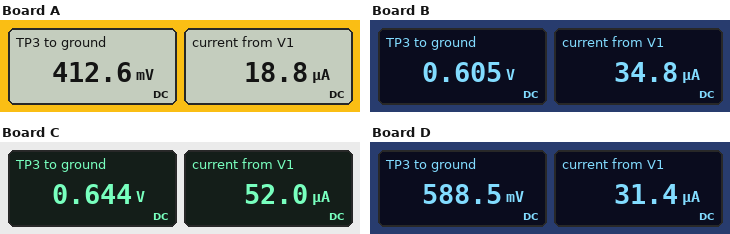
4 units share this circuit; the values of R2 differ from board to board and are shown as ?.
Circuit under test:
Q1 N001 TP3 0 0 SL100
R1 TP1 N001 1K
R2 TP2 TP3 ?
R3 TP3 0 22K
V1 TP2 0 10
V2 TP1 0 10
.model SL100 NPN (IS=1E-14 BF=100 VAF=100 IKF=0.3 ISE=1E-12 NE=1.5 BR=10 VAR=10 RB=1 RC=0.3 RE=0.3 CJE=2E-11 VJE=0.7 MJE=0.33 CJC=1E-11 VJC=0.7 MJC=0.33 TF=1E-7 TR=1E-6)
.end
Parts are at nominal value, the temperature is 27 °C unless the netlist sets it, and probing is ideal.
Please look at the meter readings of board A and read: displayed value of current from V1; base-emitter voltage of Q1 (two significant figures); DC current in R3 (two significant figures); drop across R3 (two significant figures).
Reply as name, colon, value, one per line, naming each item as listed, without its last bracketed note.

displayed value of current from V1: 18.8 µA
base-emitter voltage of Q1: 410 mV
DC current in R3: 19 µA
drop across R3: 410 mV
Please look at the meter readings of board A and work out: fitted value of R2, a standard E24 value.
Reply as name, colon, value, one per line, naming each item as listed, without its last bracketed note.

fitted value of R2, a standard E24 value: 510 kΩ
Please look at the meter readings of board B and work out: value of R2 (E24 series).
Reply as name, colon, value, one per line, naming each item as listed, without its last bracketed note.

value of R2: 270 kΩ
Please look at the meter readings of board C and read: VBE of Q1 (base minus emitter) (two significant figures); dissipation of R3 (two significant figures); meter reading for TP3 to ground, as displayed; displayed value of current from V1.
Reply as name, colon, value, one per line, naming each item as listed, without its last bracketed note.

VBE of Q1 (base minus emitter): 640 mV
dissipation of R3: 19 µW
meter reading for TP3 to ground, as displayed: 0.644 V
displayed value of current from V1: 52.0 µA
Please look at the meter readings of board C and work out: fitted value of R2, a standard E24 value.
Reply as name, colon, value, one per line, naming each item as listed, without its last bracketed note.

fitted value of R2, a standard E24 value: 180 kΩ
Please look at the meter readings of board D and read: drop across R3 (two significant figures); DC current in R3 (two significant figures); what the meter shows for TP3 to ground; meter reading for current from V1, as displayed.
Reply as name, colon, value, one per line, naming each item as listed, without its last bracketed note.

drop across R3: 590 mV
DC current in R3: 27 µA
what the meter shows for TP3 to ground: 588.5 mV
meter reading for current from V1, as displayed: 31.4 µA
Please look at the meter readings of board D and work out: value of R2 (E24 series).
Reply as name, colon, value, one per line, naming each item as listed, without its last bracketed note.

value of R2: 300 kΩ
